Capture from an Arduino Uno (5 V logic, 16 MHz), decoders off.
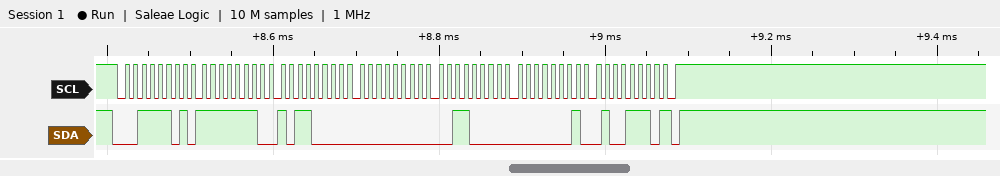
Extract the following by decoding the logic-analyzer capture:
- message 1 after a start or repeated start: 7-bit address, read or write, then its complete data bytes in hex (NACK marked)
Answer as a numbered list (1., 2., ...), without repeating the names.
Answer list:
1. 0x1E read: FE B0 00 30 01 4E NACK
